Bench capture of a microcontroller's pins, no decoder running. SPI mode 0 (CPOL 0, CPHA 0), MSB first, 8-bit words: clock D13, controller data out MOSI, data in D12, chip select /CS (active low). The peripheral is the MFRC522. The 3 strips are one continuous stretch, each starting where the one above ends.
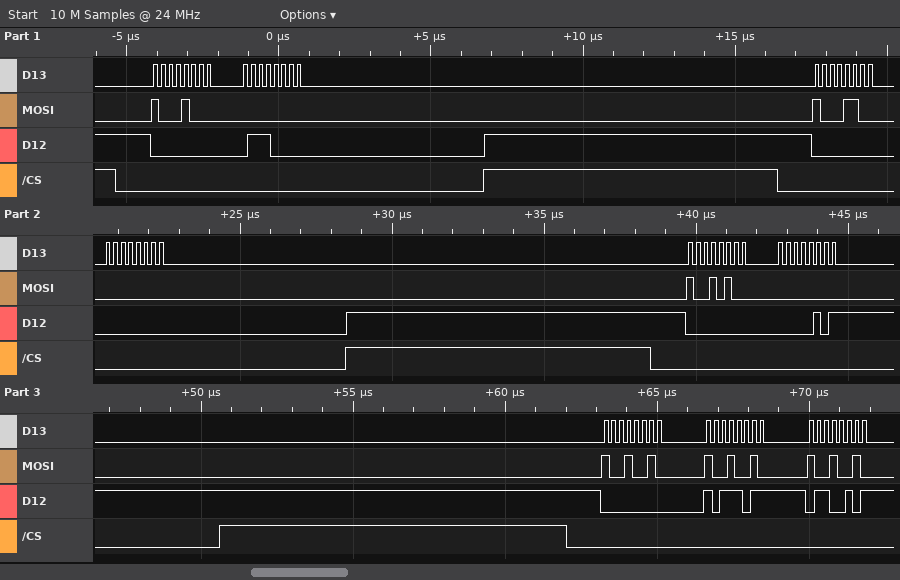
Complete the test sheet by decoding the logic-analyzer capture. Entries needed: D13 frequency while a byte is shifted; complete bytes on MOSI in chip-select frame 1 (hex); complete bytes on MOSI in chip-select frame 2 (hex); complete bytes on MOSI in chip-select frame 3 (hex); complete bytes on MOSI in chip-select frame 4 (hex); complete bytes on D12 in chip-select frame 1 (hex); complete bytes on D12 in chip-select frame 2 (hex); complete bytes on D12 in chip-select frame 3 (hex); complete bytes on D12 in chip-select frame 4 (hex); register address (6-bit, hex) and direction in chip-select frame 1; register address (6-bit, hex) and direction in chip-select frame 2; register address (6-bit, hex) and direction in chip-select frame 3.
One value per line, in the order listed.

4 MHz
88 00
8C 00
94 00
92 92 92
00 70
00 00
00 05
00 BB 65
0x04 read
0x06 read
0x0A read
